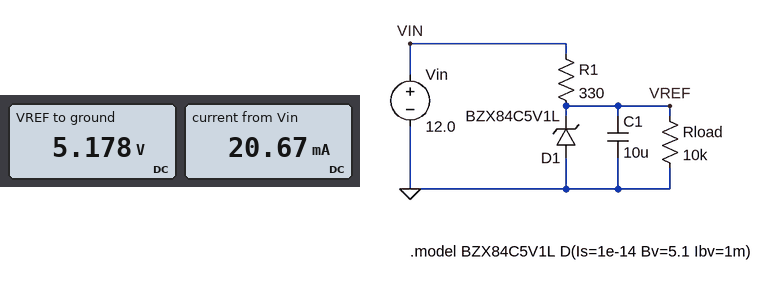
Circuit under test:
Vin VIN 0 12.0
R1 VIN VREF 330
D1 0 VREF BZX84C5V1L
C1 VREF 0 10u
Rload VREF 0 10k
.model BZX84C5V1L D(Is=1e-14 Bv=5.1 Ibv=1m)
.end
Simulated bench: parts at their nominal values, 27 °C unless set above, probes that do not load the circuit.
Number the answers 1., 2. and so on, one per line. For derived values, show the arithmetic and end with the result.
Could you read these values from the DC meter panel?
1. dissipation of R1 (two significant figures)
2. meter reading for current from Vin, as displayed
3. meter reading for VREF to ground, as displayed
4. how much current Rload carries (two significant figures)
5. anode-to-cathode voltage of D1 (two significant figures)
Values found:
1. (12 V - 5.178 V)^2 / 330 Ω = 140 mW
2. 20.67 mA
3. 5.178 V
4. (5.178 V) / 10 kΩ = 520 µA
5. 0 V - 5.178 V = -5.2 V
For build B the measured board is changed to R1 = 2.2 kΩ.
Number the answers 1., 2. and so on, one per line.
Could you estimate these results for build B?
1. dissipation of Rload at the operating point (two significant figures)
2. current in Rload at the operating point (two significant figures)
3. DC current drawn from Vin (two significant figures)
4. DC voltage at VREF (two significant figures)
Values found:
1. 2.6 mW
2. 510 µA
3. 3.1 mA
4. 5.1 V
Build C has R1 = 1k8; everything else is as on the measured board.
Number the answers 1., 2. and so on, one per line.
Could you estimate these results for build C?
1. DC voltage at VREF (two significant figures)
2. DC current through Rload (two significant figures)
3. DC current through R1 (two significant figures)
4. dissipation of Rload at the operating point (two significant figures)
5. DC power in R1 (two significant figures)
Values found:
1. 5.1 V
2. 510 µA
3. 3.8 mA
4. 2.6 mW
5. 26 mW
